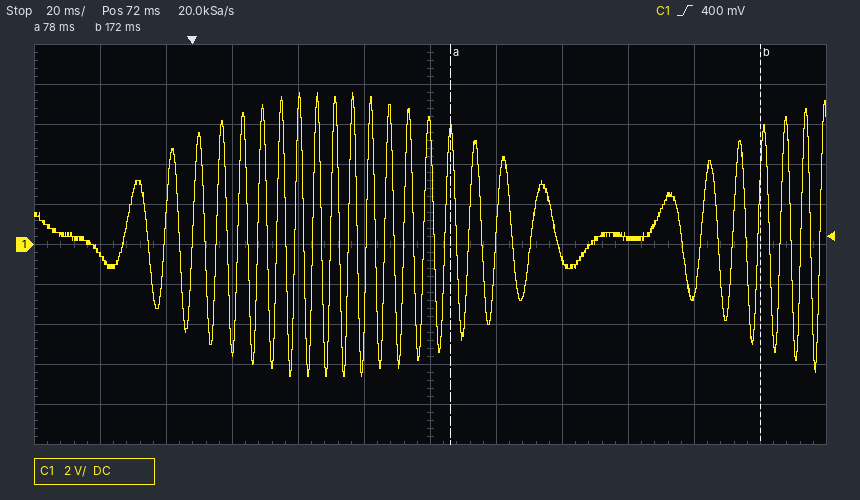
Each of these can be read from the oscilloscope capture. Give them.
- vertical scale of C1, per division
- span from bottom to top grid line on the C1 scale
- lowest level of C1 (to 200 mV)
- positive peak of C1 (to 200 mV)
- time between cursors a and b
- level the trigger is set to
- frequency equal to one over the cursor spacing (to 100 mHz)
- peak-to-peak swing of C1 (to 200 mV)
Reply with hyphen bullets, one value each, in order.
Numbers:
- 2 V
- 20 V
- -6.6 V
- 7.6 V
- 94 ms
- 400 mV
- 10.6 Hz
- 14.2 V
